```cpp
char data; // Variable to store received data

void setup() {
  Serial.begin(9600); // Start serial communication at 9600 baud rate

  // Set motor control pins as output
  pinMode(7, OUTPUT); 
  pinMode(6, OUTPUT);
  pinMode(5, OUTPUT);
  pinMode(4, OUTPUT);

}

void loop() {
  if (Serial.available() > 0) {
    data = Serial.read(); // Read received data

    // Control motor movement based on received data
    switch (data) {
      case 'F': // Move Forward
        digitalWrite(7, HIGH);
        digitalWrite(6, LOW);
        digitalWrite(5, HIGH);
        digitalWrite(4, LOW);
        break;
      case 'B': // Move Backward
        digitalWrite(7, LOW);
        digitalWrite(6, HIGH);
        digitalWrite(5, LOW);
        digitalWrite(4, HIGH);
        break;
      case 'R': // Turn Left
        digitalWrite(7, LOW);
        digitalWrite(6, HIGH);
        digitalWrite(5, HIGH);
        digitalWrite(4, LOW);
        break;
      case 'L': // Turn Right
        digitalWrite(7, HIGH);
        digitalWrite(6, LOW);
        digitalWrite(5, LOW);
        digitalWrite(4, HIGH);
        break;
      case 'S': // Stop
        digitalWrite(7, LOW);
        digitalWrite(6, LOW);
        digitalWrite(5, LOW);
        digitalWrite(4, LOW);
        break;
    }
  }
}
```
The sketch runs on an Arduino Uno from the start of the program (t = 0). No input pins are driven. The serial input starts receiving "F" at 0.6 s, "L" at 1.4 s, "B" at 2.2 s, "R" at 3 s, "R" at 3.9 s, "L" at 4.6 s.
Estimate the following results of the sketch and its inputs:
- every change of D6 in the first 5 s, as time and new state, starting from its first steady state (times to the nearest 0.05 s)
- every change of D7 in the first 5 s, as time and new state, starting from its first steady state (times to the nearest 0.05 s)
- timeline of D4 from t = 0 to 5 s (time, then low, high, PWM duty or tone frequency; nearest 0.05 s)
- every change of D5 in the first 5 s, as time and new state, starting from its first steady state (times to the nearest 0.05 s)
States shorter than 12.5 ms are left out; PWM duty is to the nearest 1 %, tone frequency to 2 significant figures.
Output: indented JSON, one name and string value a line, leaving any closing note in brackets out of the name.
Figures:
{
  "every change of D6 in the first 5 s, as time and new state, starting from its first steady state": "0 s low; 2.2 s high; 4.6 s low",
  "every change of D7 in the first 5 s, as time and new state, starting from its first steady state": "0 s low; 0.6 s high; 2.2 s low; 4.6 s high",
  "timeline of D4 from t = 0 to 5 s": "0 s low; 1.4 s high; 3 s low; 4.6 s high",
  "every change of D5 in the first 5 s, as time and new state, starting from its first steady state": "0 s low; 0.6 s high; 1.4 s low; 3 s high; 4.6 s low"
}
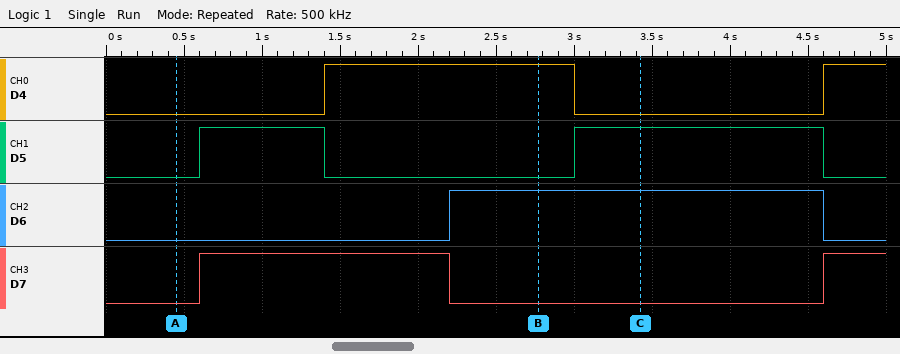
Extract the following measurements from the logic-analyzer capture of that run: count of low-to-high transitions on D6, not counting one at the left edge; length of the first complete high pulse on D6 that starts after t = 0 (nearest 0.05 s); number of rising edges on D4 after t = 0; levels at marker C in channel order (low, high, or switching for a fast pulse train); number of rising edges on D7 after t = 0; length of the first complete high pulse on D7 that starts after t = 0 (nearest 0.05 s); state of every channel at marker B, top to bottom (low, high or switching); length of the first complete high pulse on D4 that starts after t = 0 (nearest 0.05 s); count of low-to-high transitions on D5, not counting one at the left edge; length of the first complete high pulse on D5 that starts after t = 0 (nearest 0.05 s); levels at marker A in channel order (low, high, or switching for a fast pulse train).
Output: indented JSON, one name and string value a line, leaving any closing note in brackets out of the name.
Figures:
{
  "count of low-to-high transitions on D6, not counting one at the left edge": "1",
  "length of the first complete high pulse on D6 that starts after t = 0": "2.40 s",
  "number of rising edges on D4 after t = 0": "2",
  "levels at marker C in channel order": "D4 low, D5 high, D6 high, D7 low",
  "number of rising edges on D7 after t = 0": "2",
  "length of the first complete high pulse on D7 that starts after t = 0": "1.60 s",
  "state of every channel at marker B, top to bottom": "D4 high, D5 low, D6 high, D7 low",
  "length of the first complete high pulse on D4 that starts after t = 0": "1.60 s",
  "count of low-to-high transitions on D5, not counting one at the left edge": "2",
  "length of the first complete high pulse on D5 that starts after t = 0": "0.80 s",
  "levels at marker A in channel order": "D4 low, D5 low, D6 low, D7 low"
}
